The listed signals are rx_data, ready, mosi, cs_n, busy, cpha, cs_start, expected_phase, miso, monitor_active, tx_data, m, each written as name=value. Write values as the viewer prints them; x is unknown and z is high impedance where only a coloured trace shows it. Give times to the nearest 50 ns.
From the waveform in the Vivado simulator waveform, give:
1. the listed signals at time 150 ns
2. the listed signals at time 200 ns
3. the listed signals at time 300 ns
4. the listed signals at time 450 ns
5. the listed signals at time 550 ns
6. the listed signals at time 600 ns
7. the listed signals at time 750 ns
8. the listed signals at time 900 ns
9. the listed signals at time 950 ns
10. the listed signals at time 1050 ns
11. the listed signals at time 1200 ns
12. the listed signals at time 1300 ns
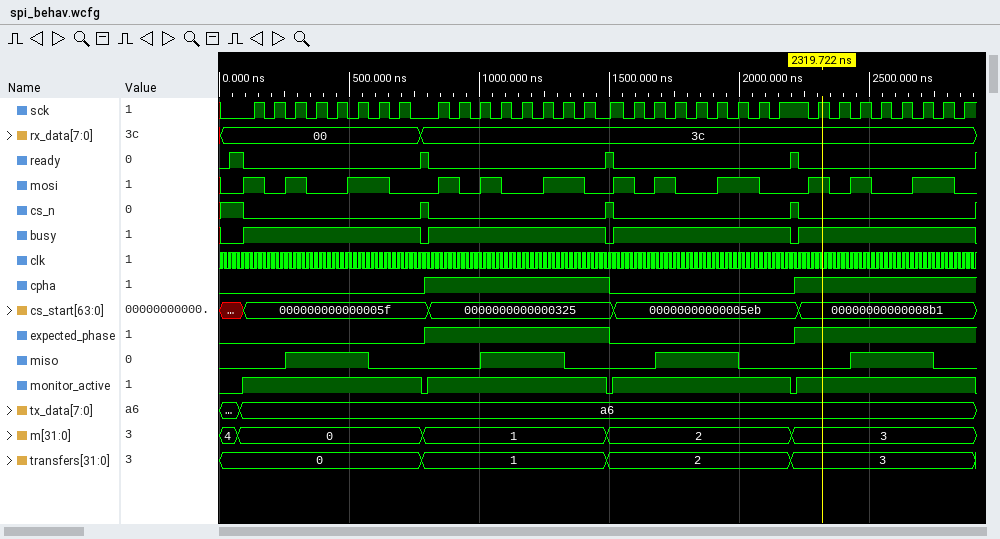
rx_data=00, ready=0, mosi=1, cs_n=0, busy=1, cpha=0, cs_start=000000000000005f, expected_phase=0, miso=0, monitor_active=1, tx_data=a6, m=0
rx_data=00, ready=0, mosi=0, cs_n=0, busy=1, cpha=0, cs_start=000000000000005f, expected_phase=0, miso=0, monitor_active=1, tx_data=a6, m=0
rx_data=00, ready=0, mosi=1, cs_n=0, busy=1, cpha=0, cs_start=000000000000005f, expected_phase=0, miso=1, monitor_active=1, tx_data=a6, m=0
rx_data=00, ready=0, mosi=0, cs_n=0, busy=1, cpha=0, cs_start=000000000000005f, expected_phase=0, miso=1, monitor_active=1, tx_data=a6, m=0
rx_data=00, ready=0, mosi=1, cs_n=0, busy=1, cpha=0, cs_start=000000000000005f, expected_phase=0, miso=1, monitor_active=1, tx_data=a6, m=0
rx_data=00, ready=0, mosi=1, cs_n=0, busy=1, cpha=0, cs_start=000000000000005f, expected_phase=0, miso=0, monitor_active=1, tx_data=a6, m=0
rx_data=00, ready=0, mosi=0, cs_n=0, busy=1, cpha=0, cs_start=000000000000005f, expected_phase=0, miso=0, monitor_active=1, tx_data=a6, m=0
rx_data=3c, ready=0, mosi=1, cs_n=0, busy=1, cpha=1, cs_start=0000000000000325, expected_phase=1, miso=0, monitor_active=1, tx_data=a6, m=1
rx_data=3c, ready=0, mosi=0, cs_n=0, busy=1, cpha=1, cs_start=0000000000000325, expected_phase=1, miso=0, monitor_active=1, tx_data=a6, m=1
rx_data=3c, ready=0, mosi=1, cs_n=0, busy=1, cpha=1, cs_start=0000000000000325, expected_phase=1, miso=1, monitor_active=1, tx_data=a6, m=1
rx_data=3c, ready=0, mosi=0, cs_n=0, busy=1, cpha=1, cs_start=0000000000000325, expected_phase=1, miso=1, monitor_active=1, tx_data=a6, m=1
rx_data=3c, ready=0, mosi=1, cs_n=0, busy=1, cpha=1, cs_start=0000000000000325, expected_phase=1, miso=1, monitor_active=1, tx_data=a6, m=1
